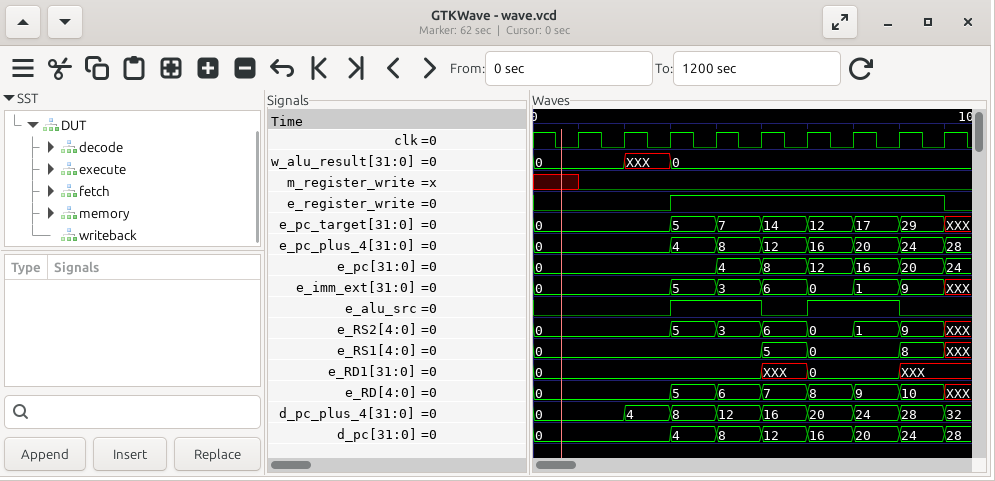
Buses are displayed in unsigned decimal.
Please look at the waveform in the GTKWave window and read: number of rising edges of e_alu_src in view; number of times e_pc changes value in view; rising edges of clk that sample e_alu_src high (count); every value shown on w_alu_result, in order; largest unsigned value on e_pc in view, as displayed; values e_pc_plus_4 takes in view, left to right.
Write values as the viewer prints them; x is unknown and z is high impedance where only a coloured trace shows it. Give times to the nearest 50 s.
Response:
2
6
4
0, XXX, 0
24
0, 4, 8, 12, 16, 20, 24, 28
